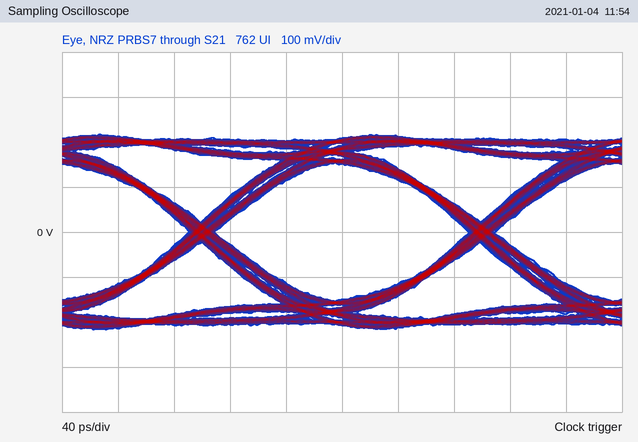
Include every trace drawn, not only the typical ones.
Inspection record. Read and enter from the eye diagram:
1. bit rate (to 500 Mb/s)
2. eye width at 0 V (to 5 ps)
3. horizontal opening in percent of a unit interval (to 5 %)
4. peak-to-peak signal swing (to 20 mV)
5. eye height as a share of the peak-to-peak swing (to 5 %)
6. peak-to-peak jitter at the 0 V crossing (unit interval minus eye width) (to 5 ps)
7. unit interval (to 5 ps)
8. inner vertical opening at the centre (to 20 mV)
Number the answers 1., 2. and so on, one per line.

1. 5.0 Gb/s
2. 180 ps
3. 90 %
4. 440 mV
5. 70 %
6. 20 ps
7. 200 ps
8. 300 mV
